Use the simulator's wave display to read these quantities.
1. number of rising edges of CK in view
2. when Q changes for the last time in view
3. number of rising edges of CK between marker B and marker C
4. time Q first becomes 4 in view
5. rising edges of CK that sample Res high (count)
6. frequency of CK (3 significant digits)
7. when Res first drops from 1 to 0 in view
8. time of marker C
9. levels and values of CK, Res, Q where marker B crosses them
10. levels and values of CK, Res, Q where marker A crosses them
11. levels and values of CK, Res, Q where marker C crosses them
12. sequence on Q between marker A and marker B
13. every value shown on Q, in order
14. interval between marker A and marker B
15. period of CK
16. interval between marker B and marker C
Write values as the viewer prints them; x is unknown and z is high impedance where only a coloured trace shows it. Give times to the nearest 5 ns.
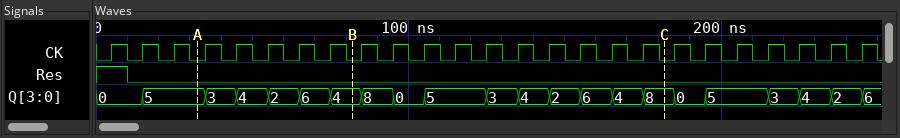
25
245 ns
10
45 ns
1
100 MHz
10 ns
180 ns
CK=0, Res=0, Q=4
CK=0, Res=0, Q=5
CK=0, Res=0, Q=8
5, 3, 4, 2, 6, 4
0, 5, 3, 4, 2, 6, 4, 8, 0, 5, 3, 4, 2, 6, 4, 8, 0, 5, 3, 4, 2, 6
50 ns
10 ns
100 ns
